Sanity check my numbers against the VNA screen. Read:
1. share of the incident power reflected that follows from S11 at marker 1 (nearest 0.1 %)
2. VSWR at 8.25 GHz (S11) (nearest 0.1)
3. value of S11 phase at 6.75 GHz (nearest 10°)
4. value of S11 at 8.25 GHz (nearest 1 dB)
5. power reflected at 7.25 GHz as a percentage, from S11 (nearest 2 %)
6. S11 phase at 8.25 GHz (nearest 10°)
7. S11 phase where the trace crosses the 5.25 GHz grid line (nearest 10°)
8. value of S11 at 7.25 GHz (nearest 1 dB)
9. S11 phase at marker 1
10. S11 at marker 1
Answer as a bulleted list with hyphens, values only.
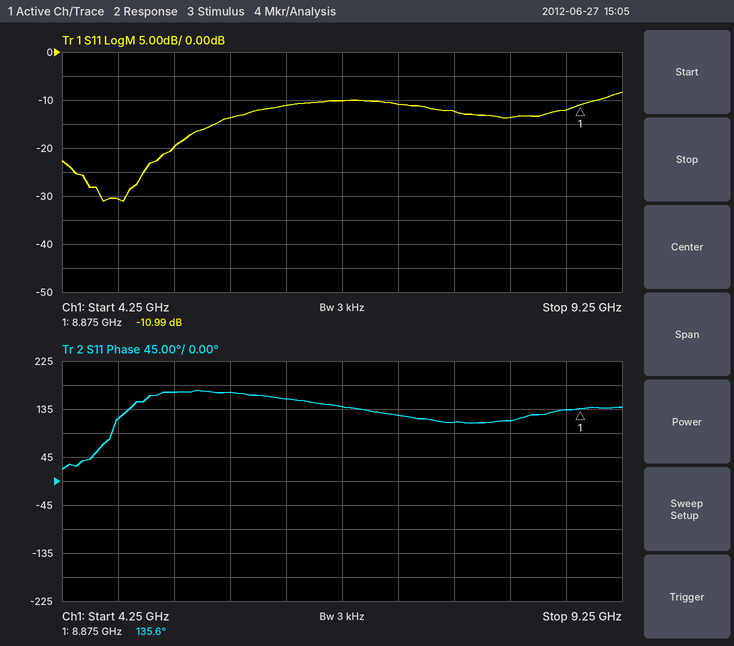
- 8.0 %
- 1.5
- 140°
- -14 dB
- 8 %
- 110°
- 170°
- -11 dB
- 135.6°
- -10.99 dB
